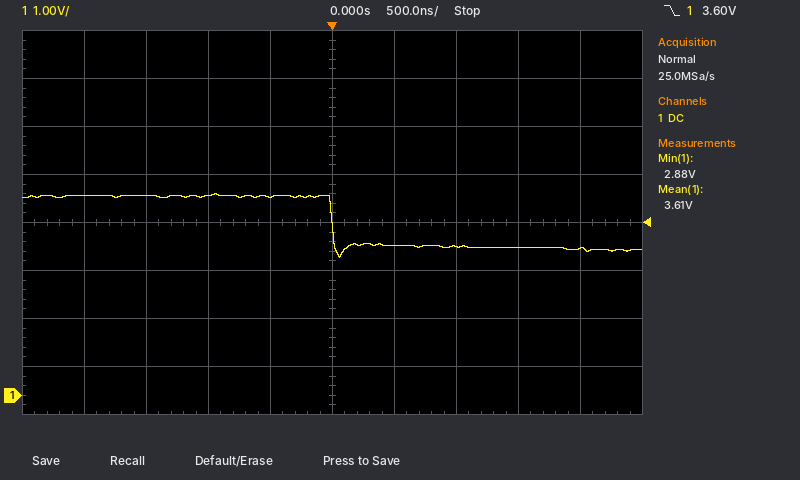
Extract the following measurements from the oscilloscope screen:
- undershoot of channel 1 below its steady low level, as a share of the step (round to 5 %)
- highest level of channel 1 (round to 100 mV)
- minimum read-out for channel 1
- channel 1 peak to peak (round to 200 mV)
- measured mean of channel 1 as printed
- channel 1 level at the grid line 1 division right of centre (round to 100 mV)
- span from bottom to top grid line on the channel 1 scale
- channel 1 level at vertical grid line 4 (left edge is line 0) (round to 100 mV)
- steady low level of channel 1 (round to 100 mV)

20 %
4.2 V
2.88 V
1.4 V
3.61 V
3.1 V
8 V
4.1 V
3.1 V
